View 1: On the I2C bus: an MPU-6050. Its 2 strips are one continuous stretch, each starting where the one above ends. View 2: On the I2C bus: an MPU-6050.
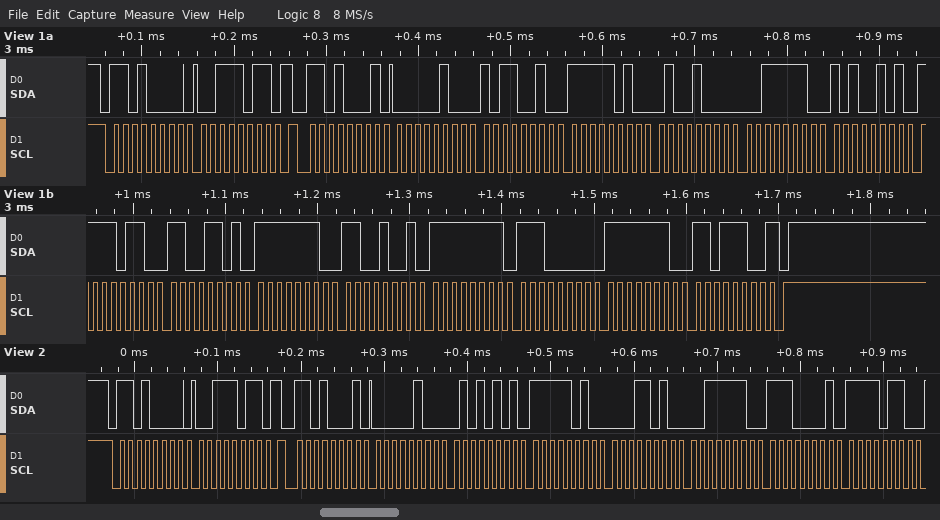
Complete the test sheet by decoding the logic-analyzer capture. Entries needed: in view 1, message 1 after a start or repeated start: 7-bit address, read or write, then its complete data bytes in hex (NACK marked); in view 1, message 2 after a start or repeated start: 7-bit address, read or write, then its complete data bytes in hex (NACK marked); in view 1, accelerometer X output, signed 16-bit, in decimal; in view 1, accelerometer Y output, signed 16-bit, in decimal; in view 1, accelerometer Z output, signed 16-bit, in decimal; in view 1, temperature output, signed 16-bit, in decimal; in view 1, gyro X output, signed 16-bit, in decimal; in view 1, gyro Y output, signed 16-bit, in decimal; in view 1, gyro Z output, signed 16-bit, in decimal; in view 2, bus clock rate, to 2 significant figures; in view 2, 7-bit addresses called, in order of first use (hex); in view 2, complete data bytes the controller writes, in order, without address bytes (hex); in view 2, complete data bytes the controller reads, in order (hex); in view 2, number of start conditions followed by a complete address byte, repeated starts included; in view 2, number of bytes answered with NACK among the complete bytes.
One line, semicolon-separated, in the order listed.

0x68 write: 3B; 0x68 read: 04 B2 FA 48 3E A5 F6 CD FE C9 FF E0 FE DC NACK; 1202; -1464; 16037; -2355; -311; -32; -292; 100 kHz; 0x68; 3B; 04 55 FA 1A 3E E1 F6; 2; 0
